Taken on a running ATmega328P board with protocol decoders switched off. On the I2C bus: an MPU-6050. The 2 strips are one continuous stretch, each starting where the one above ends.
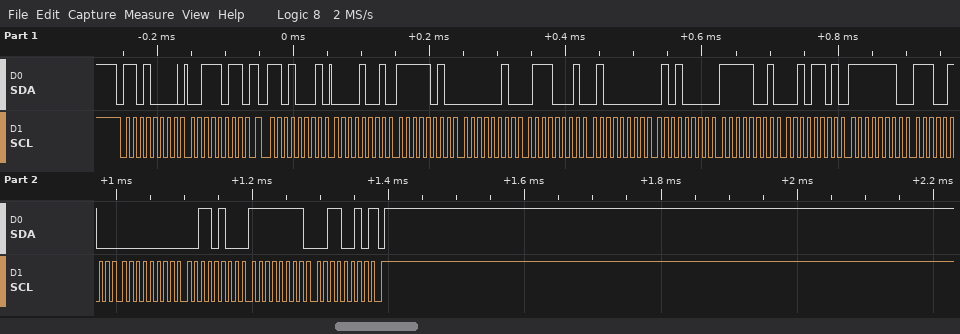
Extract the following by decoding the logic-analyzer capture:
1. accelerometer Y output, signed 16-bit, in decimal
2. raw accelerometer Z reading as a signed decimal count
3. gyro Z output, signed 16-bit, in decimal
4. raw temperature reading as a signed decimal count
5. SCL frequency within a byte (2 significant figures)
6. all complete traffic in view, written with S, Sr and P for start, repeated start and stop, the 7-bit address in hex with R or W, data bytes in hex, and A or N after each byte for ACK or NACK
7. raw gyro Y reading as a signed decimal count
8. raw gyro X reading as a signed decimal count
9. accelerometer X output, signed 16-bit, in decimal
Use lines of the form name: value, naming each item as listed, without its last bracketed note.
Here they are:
accelerometer Y output, signed 16-bit, in decimal: 625
raw accelerometer Z reading as a signed decimal count: 16464
gyro Z output, signed 16-bit, in decimal: -206
raw temperature reading as a signed decimal count: -1747
SCL frequency within a byte: 100 kHz
all complete traffic in view, written with S, Sr and P for start, repeated start and stop, the 7-bit address in hex with R or W, data bytes in hex, and A or N after each byte for ACK or NACK: S 68W A 3B A Sr 68R A 09 A FA A 02 A 71 A 40 A 50 A F9 A 2D A FE A E4 A 00 A 34 A FF A 32 N P
raw gyro Y reading as a signed decimal count: 52
raw gyro X reading as a signed decimal count: -284
accelerometer X output, signed 16-bit, in decimal: 2554
